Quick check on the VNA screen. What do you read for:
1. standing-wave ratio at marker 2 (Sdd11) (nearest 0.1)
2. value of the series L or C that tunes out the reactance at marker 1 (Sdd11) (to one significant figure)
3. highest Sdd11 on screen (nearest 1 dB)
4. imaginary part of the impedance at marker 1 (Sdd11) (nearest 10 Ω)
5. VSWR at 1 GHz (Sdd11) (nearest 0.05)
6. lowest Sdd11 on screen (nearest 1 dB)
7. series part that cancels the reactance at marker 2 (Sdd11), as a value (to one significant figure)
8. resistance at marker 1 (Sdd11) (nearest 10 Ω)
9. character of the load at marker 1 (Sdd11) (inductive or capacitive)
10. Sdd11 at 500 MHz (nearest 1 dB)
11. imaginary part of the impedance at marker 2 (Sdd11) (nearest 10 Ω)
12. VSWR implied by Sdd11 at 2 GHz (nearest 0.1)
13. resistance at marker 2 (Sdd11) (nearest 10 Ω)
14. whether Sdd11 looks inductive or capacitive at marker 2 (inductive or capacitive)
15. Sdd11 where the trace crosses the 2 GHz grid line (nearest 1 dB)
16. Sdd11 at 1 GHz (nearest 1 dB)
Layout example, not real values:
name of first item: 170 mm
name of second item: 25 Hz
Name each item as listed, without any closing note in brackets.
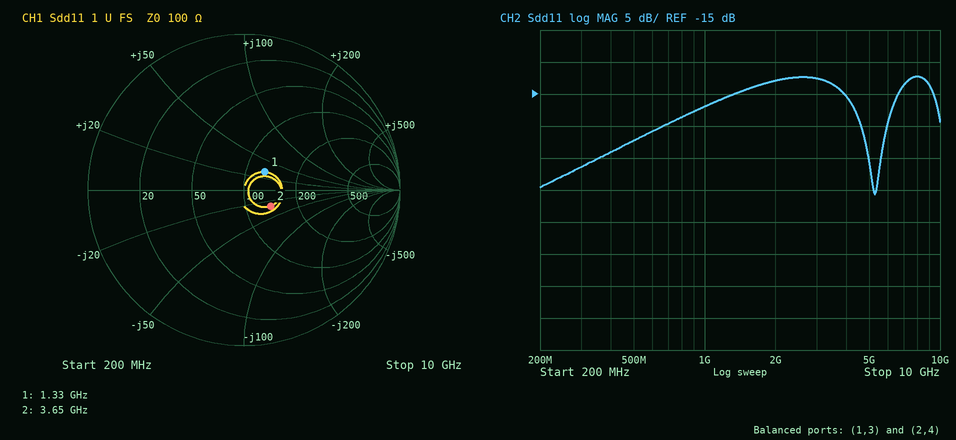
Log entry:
standing-wave ratio at marker 2 (Sdd11): 1.5
value of the series L or C that tunes out the reactance at marker 1 (Sdd11): 4 pF
highest Sdd11 on screen: -12 dB
imaginary part of the impedance at marker 1 (Sdd11): +30 Ω
VSWR at 1 GHz (Sdd11): 1.35
lowest Sdd11 on screen: -31 dB
series part that cancels the reactance at marker 2 (Sdd11), as a value: 1 nH
resistance at marker 1 (Sdd11): 130 Ω
character of the load at marker 1 (Sdd11): inductive
Sdd11 at 500 MHz: -22 dB
imaginary part of the impedance at marker 2 (Sdd11): -30 Ω
VSWR implied by Sdd11 at 2 GHz: 1.6
resistance at marker 2 (Sdd11): 140 Ω
whether Sdd11 looks inductive or capacitive at marker 2: capacitive
Sdd11 where the trace crosses the 2 GHz grid line: -13 dB
Sdd11 at 1 GHz: -17 dB
